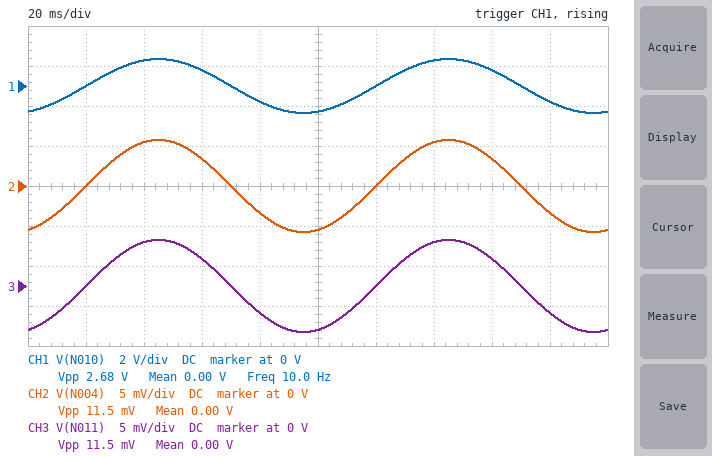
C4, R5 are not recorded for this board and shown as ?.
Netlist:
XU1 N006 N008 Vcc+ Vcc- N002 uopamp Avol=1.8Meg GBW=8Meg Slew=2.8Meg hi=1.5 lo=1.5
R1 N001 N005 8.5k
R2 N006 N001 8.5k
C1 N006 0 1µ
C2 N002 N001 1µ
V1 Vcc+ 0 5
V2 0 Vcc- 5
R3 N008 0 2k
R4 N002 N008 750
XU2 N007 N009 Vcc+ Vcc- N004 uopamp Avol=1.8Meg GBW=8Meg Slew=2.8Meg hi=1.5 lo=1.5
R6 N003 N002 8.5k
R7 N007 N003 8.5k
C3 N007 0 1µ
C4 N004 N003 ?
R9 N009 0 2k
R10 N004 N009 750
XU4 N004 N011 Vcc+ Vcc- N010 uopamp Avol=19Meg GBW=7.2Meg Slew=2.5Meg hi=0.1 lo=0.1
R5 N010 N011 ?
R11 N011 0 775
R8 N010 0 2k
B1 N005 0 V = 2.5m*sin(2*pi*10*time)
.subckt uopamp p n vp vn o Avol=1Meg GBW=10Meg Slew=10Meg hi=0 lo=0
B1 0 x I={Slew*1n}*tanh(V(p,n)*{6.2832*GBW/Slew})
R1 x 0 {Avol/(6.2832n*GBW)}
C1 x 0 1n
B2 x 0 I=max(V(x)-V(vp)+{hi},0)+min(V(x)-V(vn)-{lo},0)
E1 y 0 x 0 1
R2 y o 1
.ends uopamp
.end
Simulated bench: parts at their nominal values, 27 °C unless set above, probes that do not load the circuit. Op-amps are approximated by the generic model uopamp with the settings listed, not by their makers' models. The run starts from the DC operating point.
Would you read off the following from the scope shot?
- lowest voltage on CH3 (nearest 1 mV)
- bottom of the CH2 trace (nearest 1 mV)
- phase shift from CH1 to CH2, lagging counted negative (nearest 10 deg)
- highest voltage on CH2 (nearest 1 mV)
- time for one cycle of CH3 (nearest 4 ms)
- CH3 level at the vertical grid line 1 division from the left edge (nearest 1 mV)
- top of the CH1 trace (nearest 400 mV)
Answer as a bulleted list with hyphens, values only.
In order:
- -6 mV
- -6 mV
- 0 deg
- 6 mV
- 100 ms
- 0 V
- 1.2 V
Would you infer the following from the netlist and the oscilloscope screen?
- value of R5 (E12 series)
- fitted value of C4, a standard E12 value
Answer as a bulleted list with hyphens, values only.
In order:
- 180 kΩ
- 2.2 µF
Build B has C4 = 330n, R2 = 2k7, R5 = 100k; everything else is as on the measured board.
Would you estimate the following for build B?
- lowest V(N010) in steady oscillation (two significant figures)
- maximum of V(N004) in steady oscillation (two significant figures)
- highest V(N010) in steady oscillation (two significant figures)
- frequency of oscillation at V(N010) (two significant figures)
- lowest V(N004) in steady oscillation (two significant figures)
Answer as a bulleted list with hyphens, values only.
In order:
- -440 mV
- 3.4 mV
- 440 mV
- 10 Hz
- -3.4 mV
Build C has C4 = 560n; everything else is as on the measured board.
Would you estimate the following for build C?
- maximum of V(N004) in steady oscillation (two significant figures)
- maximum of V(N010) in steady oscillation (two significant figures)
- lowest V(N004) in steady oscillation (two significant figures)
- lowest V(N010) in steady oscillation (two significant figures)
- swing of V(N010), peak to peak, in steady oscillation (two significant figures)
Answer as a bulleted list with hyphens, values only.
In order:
- 3.3 mV
- 770 mV
- -3.3 mV
- -770 mV
- 1.5 V
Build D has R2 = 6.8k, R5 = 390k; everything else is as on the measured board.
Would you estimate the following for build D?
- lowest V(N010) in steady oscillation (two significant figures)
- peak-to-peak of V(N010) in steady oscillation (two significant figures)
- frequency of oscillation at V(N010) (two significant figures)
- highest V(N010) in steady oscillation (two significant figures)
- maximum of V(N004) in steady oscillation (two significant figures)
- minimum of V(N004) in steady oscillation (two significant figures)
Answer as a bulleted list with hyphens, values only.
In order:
- -3.0 V
- 6.0 V
- 10 Hz
- 3.0 V
- 6.0 mV
- -6.0 mV
